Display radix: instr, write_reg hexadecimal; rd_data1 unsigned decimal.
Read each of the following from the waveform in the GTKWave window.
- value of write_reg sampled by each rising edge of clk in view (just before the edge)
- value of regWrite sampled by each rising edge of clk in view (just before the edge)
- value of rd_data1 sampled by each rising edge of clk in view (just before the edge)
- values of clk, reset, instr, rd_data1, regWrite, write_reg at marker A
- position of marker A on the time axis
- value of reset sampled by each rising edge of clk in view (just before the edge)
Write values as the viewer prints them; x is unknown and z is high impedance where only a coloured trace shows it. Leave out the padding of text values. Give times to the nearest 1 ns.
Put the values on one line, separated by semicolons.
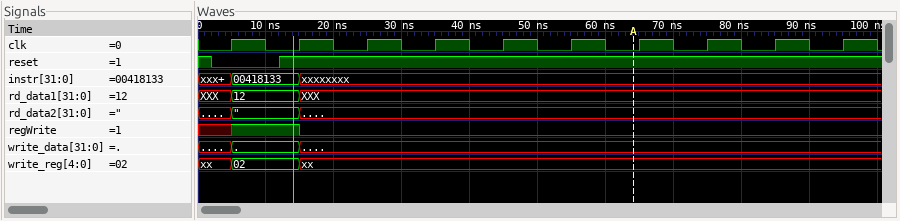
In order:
xx, 02, xx, xx, xx, xx, xx, xx, xx, xx; x 1 0 0 0 0 0 0 0 0; XXX, 12, XXX, XXX, XXX, XXX, XXX, XXX, XXX, XXX; clk=0, reset=1, instr=xxxxxxxx, rd_data1=XXX, regWrite=0, write_reg=xx; 64 ns; 0 1 1 1 1 1 1 1 1 1
